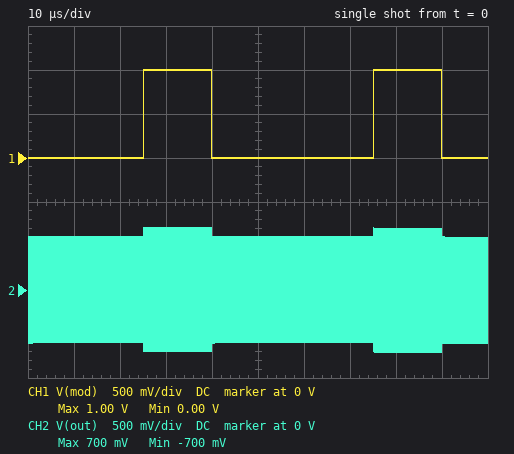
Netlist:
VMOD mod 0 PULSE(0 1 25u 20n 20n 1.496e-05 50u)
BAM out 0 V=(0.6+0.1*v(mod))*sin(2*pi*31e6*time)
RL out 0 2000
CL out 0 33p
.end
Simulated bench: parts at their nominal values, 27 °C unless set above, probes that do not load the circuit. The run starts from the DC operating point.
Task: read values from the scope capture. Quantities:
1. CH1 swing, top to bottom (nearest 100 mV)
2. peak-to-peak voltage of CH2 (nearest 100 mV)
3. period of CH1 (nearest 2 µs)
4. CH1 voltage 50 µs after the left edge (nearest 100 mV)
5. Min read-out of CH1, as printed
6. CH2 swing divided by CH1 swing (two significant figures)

1.0 V
1.4 V
50 µs
0 V
0.00 V
1.4
